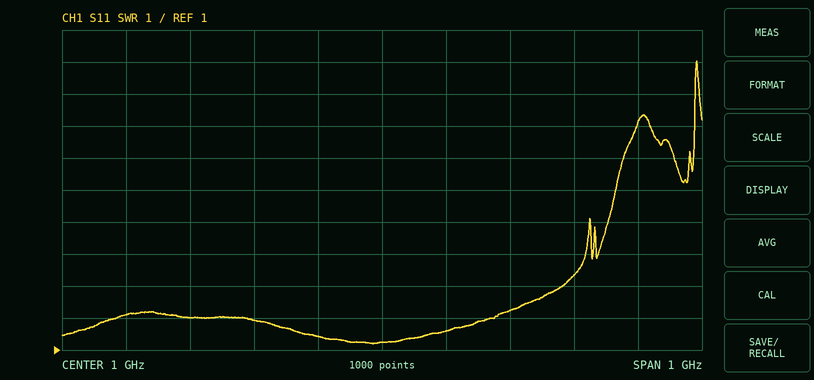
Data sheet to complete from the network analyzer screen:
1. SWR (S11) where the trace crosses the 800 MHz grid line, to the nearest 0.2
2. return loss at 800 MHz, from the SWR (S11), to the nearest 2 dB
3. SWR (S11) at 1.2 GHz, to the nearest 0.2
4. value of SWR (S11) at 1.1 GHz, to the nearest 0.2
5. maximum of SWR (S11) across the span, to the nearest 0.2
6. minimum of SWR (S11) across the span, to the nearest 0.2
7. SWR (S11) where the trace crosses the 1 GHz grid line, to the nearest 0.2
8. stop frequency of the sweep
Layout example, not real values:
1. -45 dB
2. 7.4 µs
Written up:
1. 2.0
2. 10 dB
3. 2.2
4. 1.6
5. 10.0
6. 1.2
7. 1.2
8. 1.5 GHz
